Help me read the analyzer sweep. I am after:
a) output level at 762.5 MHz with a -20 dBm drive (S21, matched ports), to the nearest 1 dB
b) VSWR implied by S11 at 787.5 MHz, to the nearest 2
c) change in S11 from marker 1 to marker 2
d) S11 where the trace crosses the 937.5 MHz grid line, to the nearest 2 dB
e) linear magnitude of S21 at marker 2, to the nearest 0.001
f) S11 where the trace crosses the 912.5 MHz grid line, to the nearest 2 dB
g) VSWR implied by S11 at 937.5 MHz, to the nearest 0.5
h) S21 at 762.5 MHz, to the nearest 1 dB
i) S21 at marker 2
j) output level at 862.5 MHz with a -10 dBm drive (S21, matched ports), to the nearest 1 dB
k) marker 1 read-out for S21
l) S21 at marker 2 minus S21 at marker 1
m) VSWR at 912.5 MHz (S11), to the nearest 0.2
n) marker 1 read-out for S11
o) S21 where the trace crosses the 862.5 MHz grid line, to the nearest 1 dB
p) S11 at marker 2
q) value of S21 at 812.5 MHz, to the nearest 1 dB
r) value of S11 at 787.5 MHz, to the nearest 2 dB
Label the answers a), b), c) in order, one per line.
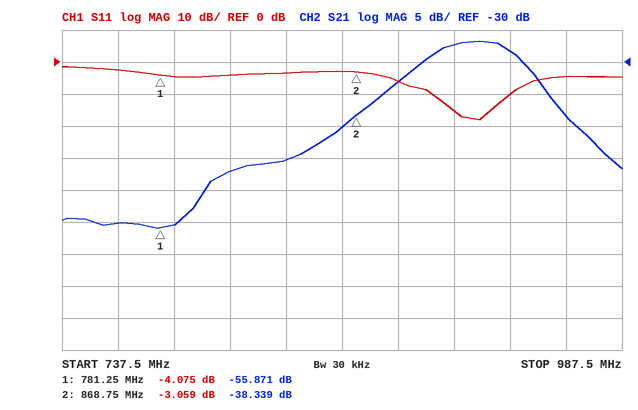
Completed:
a) -75 dBm
b) 4
c) 1.016 dB
d) -10 dB
e) 0.012
f) -16 dB
g) 2.0
h) -55 dB
i) -38.339 dB
j) -50 dBm
k) -55.871 dB
l) 17.532 dB
m) 1.4
n) -4.075 dB
o) -40 dB
p) -3.059 dB
q) -47 dB
r) -4 dB
